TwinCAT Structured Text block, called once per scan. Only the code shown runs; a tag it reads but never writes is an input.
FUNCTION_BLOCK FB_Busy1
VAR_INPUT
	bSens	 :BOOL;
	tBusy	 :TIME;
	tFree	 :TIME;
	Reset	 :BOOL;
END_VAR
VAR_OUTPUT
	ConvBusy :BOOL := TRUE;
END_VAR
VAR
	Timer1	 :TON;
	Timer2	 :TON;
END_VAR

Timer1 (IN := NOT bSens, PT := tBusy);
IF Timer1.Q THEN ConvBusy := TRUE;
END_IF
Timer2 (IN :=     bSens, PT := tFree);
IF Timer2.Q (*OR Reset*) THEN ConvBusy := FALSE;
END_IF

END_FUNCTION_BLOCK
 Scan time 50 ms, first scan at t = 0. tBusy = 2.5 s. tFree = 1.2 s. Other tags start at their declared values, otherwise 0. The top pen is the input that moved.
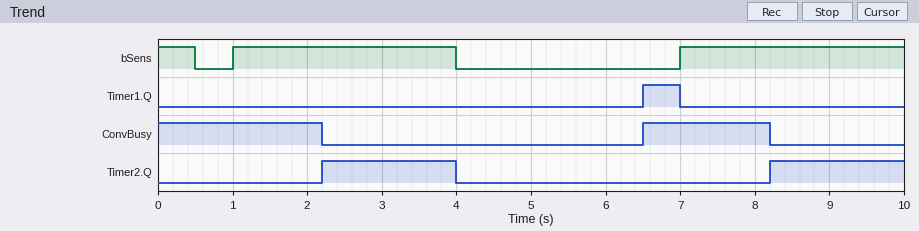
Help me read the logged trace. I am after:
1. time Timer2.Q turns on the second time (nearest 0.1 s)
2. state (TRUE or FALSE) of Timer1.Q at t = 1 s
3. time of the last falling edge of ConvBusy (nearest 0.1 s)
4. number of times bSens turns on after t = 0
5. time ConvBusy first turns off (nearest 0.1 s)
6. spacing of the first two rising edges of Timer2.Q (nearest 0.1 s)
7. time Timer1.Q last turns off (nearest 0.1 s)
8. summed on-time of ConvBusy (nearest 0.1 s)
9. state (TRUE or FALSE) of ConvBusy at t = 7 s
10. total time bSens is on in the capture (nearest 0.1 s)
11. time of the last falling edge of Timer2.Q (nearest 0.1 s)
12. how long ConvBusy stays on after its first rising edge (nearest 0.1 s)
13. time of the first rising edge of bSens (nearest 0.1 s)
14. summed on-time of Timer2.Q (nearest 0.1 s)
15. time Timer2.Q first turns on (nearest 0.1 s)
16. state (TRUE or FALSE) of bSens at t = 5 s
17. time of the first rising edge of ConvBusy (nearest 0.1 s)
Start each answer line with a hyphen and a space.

- 8.2 s
- FALSE
- 8.2 s
- 2
- 2.2 s
- 6.0 s
- 7.0 s
- 3.9 s
- TRUE
- 6.5 s
- 4.0 s
- 1.7 s
- 1.0 s
- 3.6 s
- 2.2 s
- FALSE
- 6.5 s
